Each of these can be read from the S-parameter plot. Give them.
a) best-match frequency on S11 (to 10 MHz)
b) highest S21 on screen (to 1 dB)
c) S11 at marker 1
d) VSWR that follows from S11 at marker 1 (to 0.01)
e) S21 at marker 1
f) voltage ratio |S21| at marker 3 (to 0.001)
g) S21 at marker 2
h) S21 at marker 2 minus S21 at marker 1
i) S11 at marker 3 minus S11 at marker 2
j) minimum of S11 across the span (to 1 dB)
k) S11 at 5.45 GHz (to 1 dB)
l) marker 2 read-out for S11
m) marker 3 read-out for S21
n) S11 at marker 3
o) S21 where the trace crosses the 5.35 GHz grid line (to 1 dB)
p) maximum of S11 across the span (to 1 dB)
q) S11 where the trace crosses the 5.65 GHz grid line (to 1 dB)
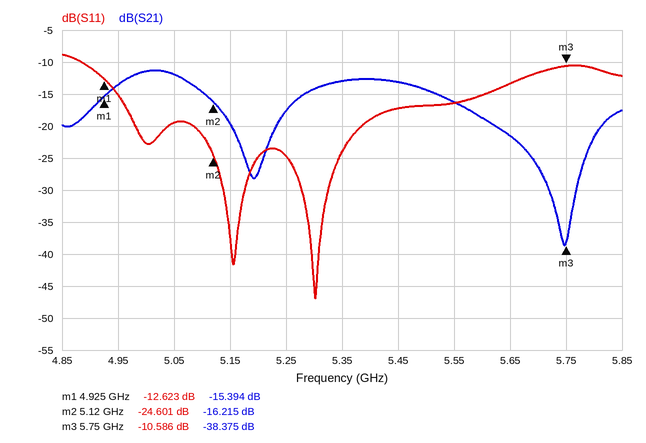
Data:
5.30 GHz
-11 dB
-12.623 dB
1.61
-15.394 dB
0.012
-16.215 dB
-0.821 dB
14.015 dB
-47 dB
-17 dB
-24.601 dB
-38.375 dB
-10.586 dB
-13 dB
-9 dB
-13 dB
